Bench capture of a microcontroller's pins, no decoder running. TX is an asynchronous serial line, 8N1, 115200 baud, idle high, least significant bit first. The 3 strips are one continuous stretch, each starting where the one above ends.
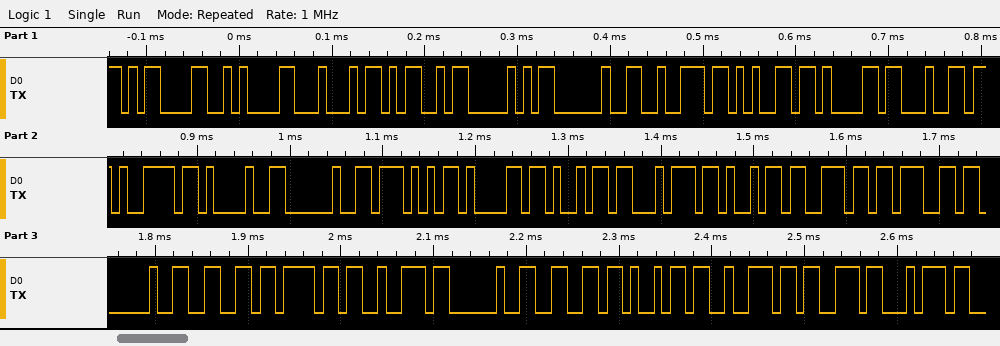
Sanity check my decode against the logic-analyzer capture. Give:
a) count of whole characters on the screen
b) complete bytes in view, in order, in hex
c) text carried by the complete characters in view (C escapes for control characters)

30
0D 0A 44 4D 50 20 72 65 61 64 79 21 20 57 61 69 74 69 6E 67 20 66 6F 72 20 66 69 72 73 74
"\r\nDMP ready! Waiting for first"
